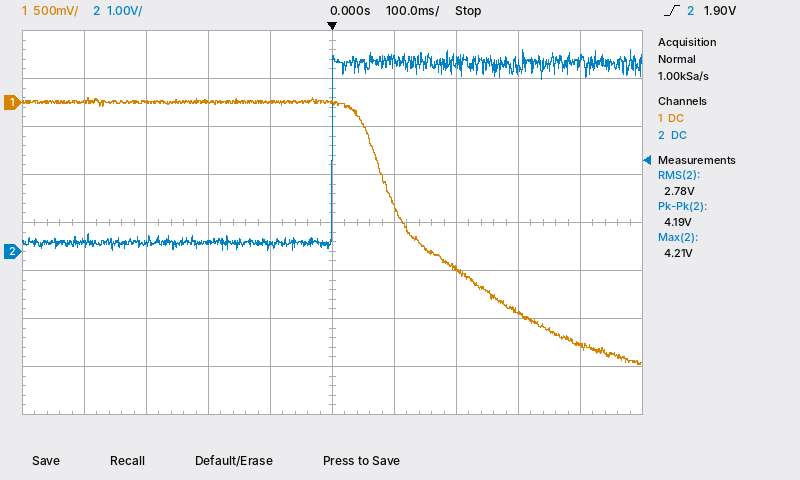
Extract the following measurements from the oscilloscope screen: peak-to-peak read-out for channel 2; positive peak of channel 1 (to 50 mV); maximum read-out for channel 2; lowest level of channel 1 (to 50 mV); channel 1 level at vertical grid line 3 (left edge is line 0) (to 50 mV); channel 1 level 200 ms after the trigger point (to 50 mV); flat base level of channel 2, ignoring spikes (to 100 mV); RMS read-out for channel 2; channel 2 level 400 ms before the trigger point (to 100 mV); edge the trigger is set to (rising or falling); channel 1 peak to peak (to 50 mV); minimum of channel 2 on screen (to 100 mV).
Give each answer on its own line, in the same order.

4.19 V
50 mV
4.21 V
-2.75 V
0 mV
-1.75 V
200 mV
2.78 V
200 mV
rising
2.80 V
0.0 V
